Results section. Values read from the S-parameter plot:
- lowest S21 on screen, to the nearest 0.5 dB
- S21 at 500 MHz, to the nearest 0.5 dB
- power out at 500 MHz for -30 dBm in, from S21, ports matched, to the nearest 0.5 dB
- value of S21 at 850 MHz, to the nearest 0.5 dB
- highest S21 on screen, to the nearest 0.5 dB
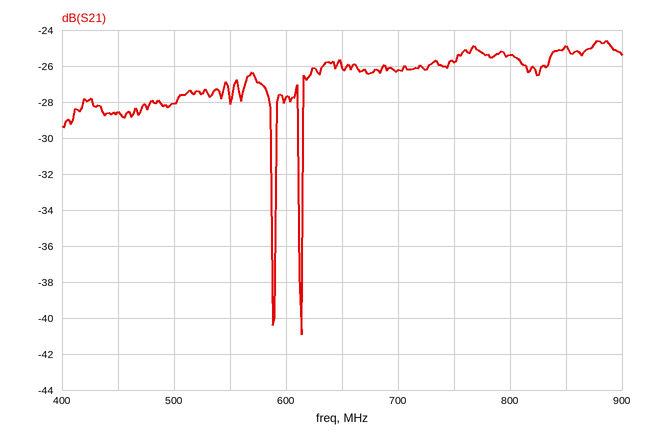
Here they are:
-41.0 dB
-28.0 dB
-58.0 dBm
-25.0 dB
-24.5 dB
